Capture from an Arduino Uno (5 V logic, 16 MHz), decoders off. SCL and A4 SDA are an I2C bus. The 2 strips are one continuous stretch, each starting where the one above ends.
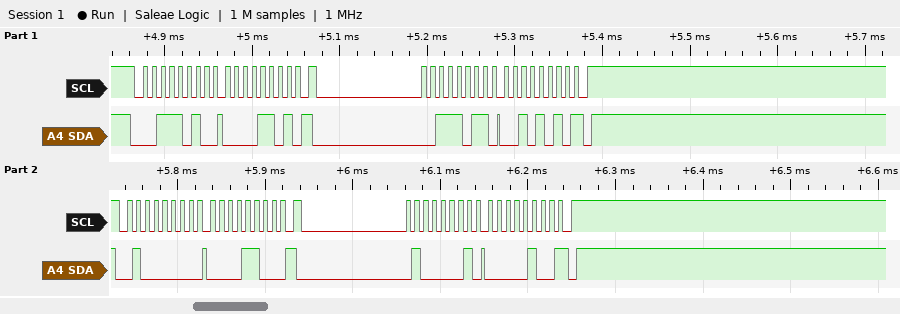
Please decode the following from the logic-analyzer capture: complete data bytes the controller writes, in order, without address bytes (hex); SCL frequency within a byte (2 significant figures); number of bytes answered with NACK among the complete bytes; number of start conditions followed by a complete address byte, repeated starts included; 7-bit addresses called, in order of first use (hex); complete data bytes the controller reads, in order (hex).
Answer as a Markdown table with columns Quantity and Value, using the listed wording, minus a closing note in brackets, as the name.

| Quantity | Value |
|---|---|
| complete data bytes the controller writes, in order, without address bytes | 0D 0C |
| SCL frequency within a byte | 100 kHz |
| number of bytes answered with NACK among the complete bytes | 2 |
| number of start conditions followed by a complete address byte, repeated starts included | 4 |
| 7-bit addresses called, in order of first use | 0x1D 0x20 |
| complete data bytes the controller reads, in order | 2A 04 |
